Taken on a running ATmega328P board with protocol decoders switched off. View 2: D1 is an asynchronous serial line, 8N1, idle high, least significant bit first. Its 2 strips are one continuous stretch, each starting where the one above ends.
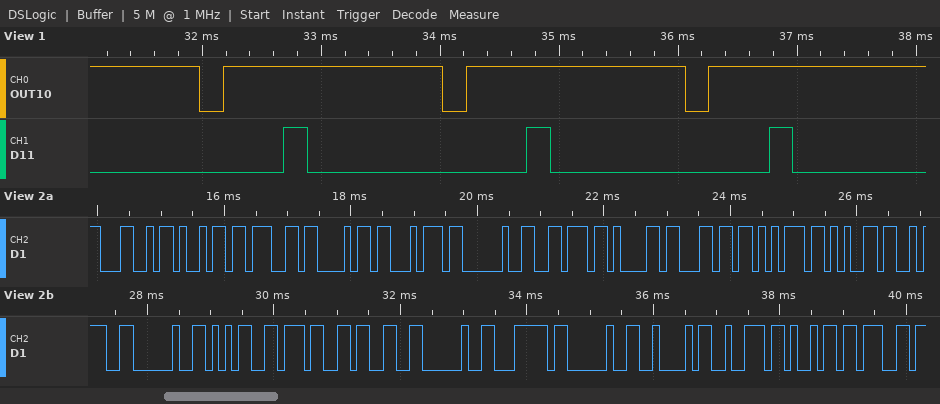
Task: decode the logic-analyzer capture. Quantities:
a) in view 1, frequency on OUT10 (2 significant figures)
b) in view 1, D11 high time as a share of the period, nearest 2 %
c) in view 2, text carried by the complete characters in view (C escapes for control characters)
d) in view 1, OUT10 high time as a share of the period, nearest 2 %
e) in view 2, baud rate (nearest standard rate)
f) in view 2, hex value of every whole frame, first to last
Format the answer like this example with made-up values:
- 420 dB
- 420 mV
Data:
- 490 Hz
- 10 %
- "Light value: 573 | Brig"
- 90 %
- 9600 baud
- 4C 69 67 68 74 20 76 61 6C 75 65 3A 20 35 37 33 20 7C 20 42 72 69 67
